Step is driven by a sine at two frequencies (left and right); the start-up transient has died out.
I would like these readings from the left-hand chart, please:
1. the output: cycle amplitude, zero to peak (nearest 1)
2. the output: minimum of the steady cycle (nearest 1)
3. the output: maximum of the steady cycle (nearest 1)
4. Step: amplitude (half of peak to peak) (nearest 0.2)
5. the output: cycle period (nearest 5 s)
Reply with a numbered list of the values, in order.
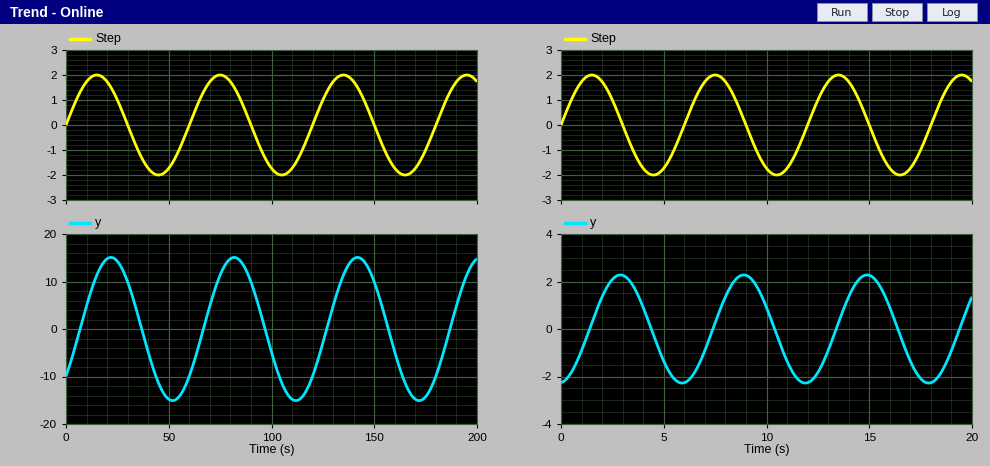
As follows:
1. 15
2. -15
3. 15
4. 2.0
5. 60 s
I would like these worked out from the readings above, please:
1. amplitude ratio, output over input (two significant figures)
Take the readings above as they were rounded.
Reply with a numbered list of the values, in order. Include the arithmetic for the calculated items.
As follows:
1. 15 / 2 = 7.5
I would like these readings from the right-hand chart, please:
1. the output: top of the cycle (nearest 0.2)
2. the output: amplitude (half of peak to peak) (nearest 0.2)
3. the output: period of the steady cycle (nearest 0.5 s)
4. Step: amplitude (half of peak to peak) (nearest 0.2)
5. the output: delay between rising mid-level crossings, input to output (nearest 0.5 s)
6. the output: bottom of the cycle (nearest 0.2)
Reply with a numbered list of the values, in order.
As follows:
1. 2.2
2. 2.2
3. 6.0 s
4. 2.0
5. 1.5 s
6. -2.2
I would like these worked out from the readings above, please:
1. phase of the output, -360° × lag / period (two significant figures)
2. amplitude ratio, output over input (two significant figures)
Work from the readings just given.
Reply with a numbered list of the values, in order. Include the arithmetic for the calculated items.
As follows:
1. -360 × 1.5 / 6 = -90°
2. 2.2 / 2 = 1.1
